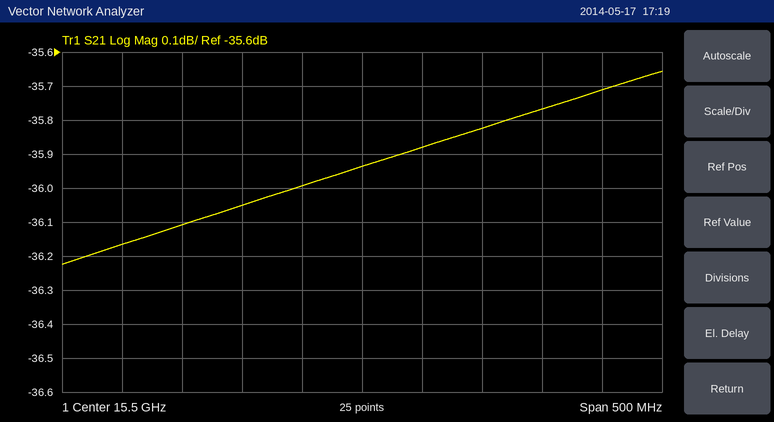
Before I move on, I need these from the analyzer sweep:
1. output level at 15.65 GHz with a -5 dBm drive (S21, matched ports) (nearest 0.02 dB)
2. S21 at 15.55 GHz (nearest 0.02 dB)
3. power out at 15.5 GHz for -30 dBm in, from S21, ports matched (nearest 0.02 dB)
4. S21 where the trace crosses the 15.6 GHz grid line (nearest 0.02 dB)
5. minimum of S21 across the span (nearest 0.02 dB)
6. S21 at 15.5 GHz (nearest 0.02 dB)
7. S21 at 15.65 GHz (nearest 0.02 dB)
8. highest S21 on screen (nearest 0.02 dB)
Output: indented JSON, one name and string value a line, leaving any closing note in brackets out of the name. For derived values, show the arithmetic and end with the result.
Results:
{
  "output level at 15.65 GHz with a -5 dBm drive (S21, matched ports)": "-5 dBm + (-35.76 dB) = -40.76 dBm",
  "S21 at 15.55 GHz": "-35.88 dB",
  "power out at 15.5 GHz for -30 dBm in, from S21, ports matched": "-30 dBm + (-35.94 dB) = -65.94 dBm",
  "S21 where the trace crosses the 15.6 GHz grid line": "-35.82 dB",
  "minimum of S21 across the span": "-36.22 dB",
  "S21 at 15.5 GHz": "-35.94 dB",
  "S21 at 15.65 GHz": "-35.76 dB",
  "highest S21 on screen": "-35.66 dB"
}
